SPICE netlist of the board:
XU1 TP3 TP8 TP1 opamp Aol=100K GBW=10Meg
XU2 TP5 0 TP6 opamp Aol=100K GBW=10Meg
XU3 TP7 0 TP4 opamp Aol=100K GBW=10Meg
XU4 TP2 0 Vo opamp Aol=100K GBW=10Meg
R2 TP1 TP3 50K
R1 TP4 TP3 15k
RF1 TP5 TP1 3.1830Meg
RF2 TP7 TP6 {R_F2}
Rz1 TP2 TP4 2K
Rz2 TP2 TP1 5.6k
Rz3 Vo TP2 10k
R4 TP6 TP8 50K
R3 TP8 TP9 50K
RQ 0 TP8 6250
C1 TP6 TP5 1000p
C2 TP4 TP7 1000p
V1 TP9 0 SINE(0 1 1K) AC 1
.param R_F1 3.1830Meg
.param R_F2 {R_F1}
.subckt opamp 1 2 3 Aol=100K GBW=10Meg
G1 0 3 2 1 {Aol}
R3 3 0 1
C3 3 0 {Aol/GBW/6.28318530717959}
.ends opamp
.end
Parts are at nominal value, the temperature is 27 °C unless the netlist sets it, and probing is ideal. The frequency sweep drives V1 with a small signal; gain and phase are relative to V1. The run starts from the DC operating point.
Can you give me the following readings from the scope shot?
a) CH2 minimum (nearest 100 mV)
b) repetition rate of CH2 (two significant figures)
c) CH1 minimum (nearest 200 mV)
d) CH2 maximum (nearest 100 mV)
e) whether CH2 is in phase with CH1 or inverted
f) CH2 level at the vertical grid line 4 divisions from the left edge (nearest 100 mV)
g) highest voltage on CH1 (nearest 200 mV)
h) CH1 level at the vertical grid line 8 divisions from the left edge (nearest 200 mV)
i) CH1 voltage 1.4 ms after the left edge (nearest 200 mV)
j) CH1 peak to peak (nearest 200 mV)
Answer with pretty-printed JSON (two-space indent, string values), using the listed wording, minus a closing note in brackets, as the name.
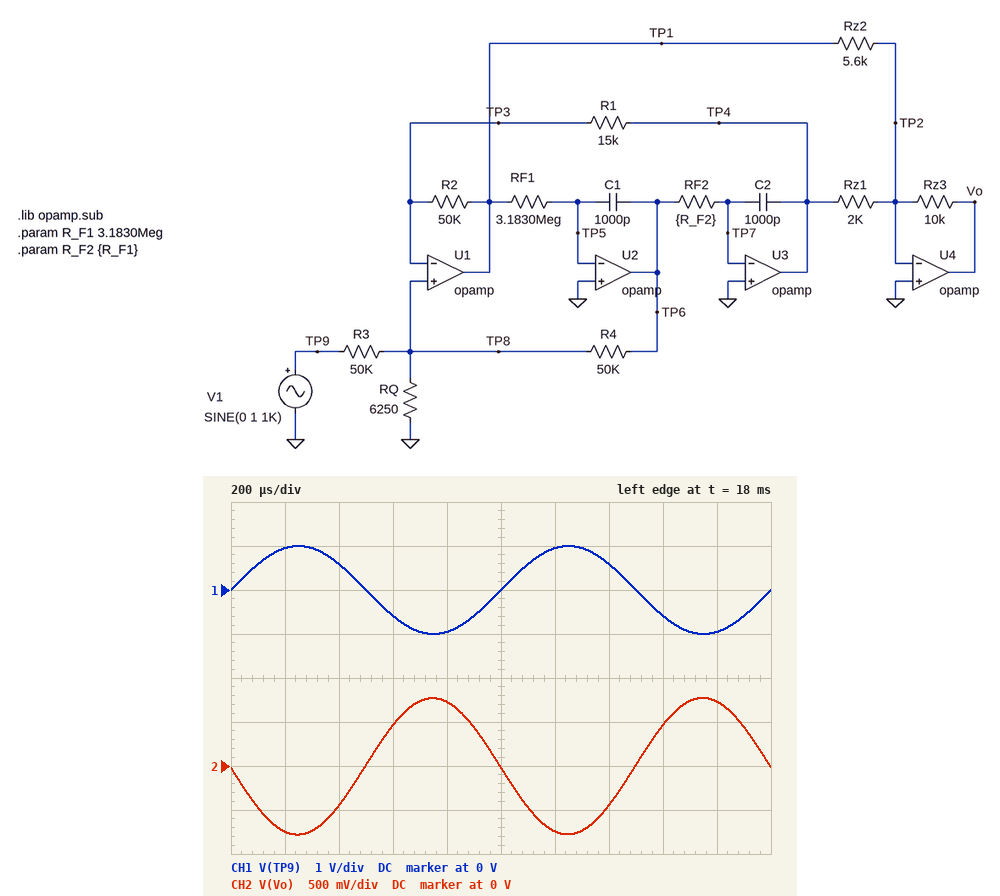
{
  "CH2 minimum": "-800 mV",
  "repetition rate of CH2": "1.0 kHz",
  "CH1 minimum": "-1.0 V",
  "CH2 maximum": "800 mV",
  "whether CH2 is in phase with CH1 or inverted": "inverted",
  "CH2 level at the vertical grid line 4 divisions from the left edge": "700 mV",
  "highest voltage on CH1": "1.0 V",
  "CH1 level at the vertical grid line 8 divisions from the left edge": "-600 mV",
  "CH1 voltage 1.4 ms after the left edge": "600 mV",
  "CH1 peak to peak": "2.0 V"
}
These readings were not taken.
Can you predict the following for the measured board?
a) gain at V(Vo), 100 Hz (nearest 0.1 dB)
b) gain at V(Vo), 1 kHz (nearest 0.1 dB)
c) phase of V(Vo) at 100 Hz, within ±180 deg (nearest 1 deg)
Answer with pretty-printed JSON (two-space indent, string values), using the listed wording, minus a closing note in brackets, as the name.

{
  "gain at V(Vo), 100 Hz": "-1.4 dB",
  "gain at V(Vo), 1 kHz": "-2.2 dB",
  "phase of V(Vo) at 100 Hz, within ±180 deg": "-128 deg"
}
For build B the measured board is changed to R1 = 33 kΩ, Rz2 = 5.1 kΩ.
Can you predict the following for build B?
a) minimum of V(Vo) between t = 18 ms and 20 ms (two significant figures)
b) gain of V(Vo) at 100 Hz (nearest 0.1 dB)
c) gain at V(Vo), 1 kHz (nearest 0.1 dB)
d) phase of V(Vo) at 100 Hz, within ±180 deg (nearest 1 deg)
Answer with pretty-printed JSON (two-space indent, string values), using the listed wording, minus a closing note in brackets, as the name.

{
  "minimum of V(Vo) between t = 18 ms and 20 ms": "-500 mV",
  "gain of V(Vo) at 100 Hz": "-11.0 dB",
  "gain at V(Vo), 1 kHz": "-6.2 dB",
  "phase of V(Vo) at 100 Hz, within ±180 deg": "-169 deg"
}
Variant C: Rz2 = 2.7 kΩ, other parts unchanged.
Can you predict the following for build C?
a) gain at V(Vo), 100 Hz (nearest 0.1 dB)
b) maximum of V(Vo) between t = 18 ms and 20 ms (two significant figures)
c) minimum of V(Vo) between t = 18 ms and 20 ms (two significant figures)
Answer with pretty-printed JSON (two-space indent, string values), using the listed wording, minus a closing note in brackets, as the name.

{
  "gain at V(Vo), 100 Hz": "11.8 dB",
  "maximum of V(Vo) between t = 18 ms and 20 ms": "1.6 V",
  "minimum of V(Vo) between t = 18 ms and 20 ms": "-1.6 V"
}
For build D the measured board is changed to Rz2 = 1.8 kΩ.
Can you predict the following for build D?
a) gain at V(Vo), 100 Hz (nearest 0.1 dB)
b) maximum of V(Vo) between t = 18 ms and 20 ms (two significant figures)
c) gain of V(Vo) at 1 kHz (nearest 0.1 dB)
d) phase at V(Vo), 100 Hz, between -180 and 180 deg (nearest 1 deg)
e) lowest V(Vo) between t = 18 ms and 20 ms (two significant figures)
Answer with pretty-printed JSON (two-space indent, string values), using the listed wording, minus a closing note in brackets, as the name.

{
  "gain at V(Vo), 100 Hz": "16.7 dB",
  "maximum of V(Vo) between t = 18 ms and 20 ms": "2.4 V",
  "gain of V(Vo) at 1 kHz": "7.7 dB",
  "phase at V(Vo), 100 Hz, between -180 and 180 deg": "-128 deg",
  "lowest V(Vo) between t = 18 ms and 20 ms": "-2.5 V"
}
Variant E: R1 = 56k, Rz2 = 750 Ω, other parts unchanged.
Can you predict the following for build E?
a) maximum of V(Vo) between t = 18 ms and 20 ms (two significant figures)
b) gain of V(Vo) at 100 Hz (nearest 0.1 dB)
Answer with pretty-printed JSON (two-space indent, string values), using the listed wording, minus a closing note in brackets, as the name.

{
  "maximum of V(Vo) between t = 18 ms and 20 ms": "2.5 V",
  "gain of V(Vo) at 100 Hz": "9.3 dB"
}
